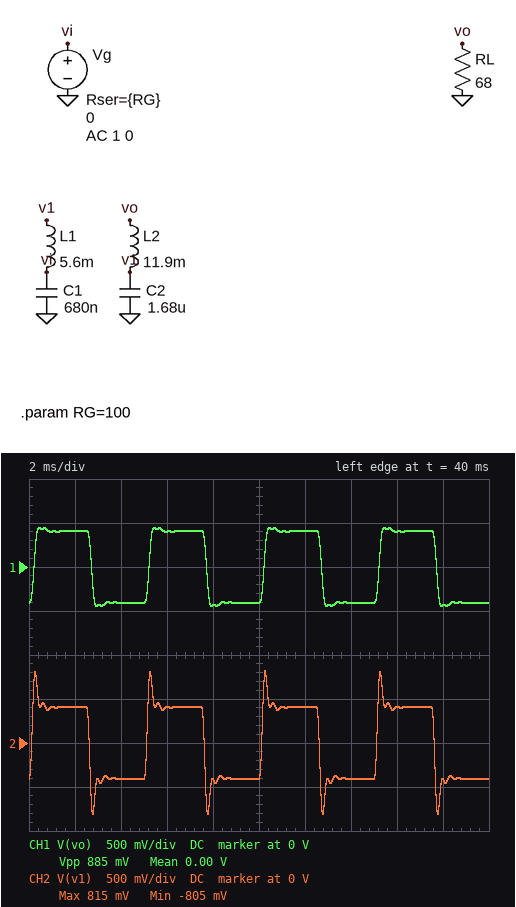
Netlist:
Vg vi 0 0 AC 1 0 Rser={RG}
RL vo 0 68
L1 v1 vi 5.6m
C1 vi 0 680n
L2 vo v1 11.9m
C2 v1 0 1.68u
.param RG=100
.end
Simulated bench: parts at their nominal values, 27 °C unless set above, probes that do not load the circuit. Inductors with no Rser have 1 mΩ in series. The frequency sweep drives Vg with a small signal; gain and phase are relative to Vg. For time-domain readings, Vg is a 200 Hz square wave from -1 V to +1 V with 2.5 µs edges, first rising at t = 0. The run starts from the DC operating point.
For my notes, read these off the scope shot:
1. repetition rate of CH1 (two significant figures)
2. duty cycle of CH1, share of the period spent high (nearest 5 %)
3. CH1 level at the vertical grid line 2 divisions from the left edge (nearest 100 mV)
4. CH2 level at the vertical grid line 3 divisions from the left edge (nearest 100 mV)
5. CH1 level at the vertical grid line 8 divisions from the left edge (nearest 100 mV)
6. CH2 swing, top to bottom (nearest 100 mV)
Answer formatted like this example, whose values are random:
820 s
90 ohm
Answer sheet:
200 Hz
50 %
-400 mV
400 mV
400 mV
1.6 V
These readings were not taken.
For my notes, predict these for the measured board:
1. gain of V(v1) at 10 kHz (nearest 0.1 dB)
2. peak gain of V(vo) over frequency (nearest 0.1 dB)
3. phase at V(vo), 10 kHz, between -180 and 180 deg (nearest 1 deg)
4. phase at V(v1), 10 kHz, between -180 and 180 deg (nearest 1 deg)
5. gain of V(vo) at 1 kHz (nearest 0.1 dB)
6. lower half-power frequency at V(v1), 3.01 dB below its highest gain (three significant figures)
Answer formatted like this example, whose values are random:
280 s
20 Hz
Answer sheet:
-43.3 dB
-7.7 dB
19 deg
104 deg
-8.2 dB
344 Hz
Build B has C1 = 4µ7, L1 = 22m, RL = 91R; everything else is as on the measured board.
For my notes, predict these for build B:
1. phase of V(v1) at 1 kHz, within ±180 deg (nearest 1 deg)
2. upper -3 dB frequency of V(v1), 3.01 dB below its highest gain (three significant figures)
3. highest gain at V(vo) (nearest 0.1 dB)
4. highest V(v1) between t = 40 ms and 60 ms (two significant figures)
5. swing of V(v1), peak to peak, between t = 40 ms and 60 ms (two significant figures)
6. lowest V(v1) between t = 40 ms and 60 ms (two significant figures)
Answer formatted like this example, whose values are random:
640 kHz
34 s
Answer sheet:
-127 deg
1.15 kHz
-6.4 dB
510 mV
1.0 V
-510 mV
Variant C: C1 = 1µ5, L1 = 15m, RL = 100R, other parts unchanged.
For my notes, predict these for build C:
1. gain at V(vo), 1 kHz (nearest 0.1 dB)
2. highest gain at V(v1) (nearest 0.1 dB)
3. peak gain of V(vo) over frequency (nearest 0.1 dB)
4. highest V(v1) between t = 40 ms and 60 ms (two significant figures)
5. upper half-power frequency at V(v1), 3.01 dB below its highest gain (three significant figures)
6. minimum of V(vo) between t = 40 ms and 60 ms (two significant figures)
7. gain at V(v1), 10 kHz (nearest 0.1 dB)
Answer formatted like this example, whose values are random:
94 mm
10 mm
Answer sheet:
-6.5 dB
-2.7 dB
-6.0 dB
760 mV
1.76 kHz
-620 mV
-59.2 dB
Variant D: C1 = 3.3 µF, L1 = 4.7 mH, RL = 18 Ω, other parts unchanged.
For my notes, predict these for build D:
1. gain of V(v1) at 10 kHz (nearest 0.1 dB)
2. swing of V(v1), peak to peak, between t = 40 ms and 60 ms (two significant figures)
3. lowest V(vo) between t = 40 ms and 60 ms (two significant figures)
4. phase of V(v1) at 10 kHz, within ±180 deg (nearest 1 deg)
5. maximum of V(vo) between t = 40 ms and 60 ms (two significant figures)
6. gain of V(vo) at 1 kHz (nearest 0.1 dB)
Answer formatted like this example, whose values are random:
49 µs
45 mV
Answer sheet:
-55.7 dB
1.4 V
-240 mV
93 deg
240 mV
-20.2 dB
